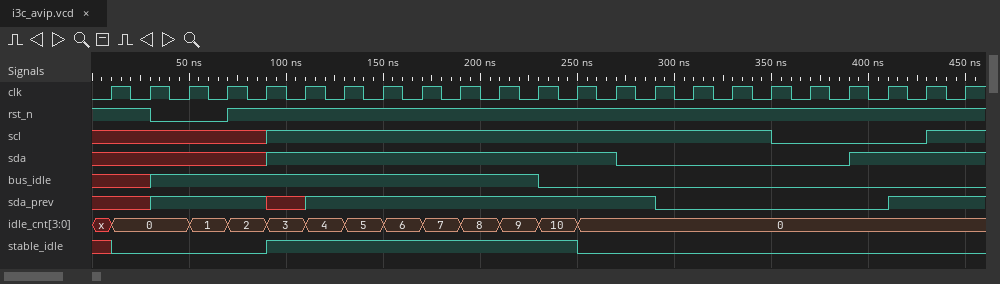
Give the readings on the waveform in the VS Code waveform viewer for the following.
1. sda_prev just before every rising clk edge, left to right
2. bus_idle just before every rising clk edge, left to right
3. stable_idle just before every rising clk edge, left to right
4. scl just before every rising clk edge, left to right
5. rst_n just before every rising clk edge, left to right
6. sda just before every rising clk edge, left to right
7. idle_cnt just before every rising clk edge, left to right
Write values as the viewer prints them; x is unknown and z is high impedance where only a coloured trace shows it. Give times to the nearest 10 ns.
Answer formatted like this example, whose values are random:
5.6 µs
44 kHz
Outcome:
x x 1 1 1 x 1 1 1 1 1 1 1 1 1 0 0 0 0 0 0 1 1
x x 1 1 1 1 1 1 1 1 1 1 0 0 0 0 0 0 0 0 0 0 0
x 0 0 0 0 1 1 1 1 1 1 1 1 0 0 0 0 0 0 0 0 0 0
x x x x x 1 1 1 1 1 1 1 1 1 1 1 1 1 0 0 0 0 1
1 1 0 0 1 1 1 1 1 1 1 1 1 1 1 1 1 1 1 1 1 1 1
x x x x x 1 1 1 1 1 1 1 1 1 0 0 0 0 0 0 1 1 1
x, 0, 0, 1, 2, 3, 4, 5, 6, 7, 8, 9, 10, 0, 0, 0, 0, 0, 0, 0, 0, 0, 0
